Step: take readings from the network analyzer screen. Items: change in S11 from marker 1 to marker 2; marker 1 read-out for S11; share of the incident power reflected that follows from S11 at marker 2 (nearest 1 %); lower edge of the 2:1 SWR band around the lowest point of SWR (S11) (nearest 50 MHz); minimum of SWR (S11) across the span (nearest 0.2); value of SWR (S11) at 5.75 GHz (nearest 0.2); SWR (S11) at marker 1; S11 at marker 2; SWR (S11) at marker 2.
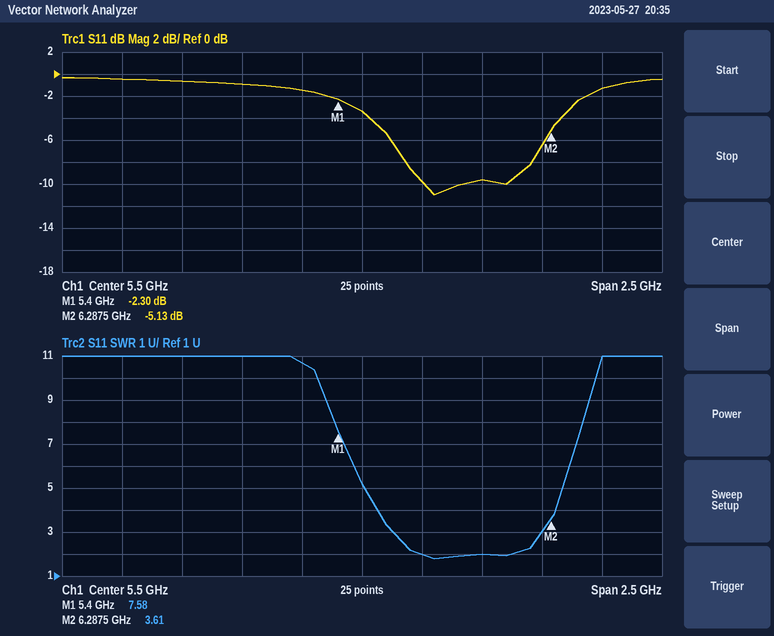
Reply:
-2.83 dB
-2.30 dB
31 %
5.75 GHz
1.8
2.0
7.58
-5.13 dB
3.61
